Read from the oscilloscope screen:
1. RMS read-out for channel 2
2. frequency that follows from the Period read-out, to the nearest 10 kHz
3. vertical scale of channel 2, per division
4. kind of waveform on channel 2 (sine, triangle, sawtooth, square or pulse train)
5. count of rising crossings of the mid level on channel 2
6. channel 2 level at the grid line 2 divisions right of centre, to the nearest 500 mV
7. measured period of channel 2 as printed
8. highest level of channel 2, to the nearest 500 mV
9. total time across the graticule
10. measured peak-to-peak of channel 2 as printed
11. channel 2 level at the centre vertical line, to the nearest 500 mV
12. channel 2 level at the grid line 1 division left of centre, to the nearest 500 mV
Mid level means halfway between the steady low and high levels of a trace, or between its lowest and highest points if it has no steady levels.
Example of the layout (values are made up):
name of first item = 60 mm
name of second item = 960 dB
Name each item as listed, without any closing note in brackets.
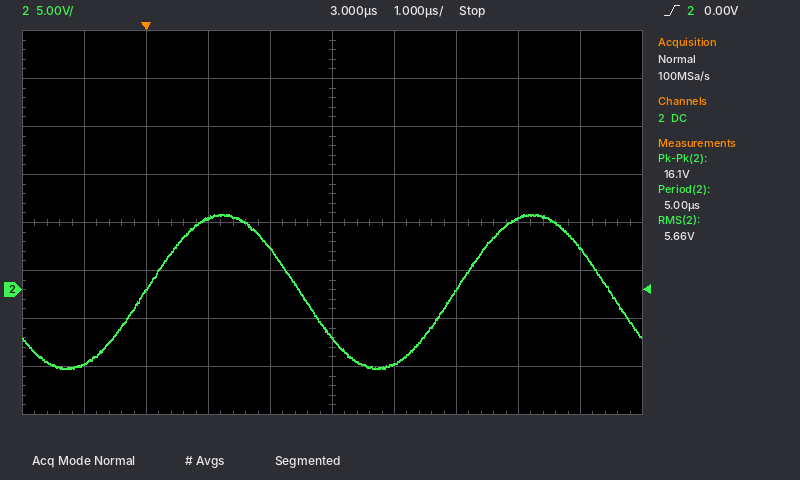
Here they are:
RMS read-out for channel 2 = 5.66 V
frequency that follows from the Period read-out, to the nearest 10 kHz = 200 kHz
vertical scale of channel 2, per division = 5 V
kind of waveform on channel 2 = sine
count of rising crossings of the mid level on channel 2 = 2
channel 2 level at the grid line 2 divisions right of centre, to the nearest 500 mV = 0.0 V
measured period of channel 2 as printed = 5.00 µs
highest level of channel 2, to the nearest 500 mV = 8.0 V
total time across the graticule = 10 µs
measured peak-to-peak of channel 2 as printed = 16.1 V
channel 2 level at the centre vertical line, to the nearest 500 mV = -5.0 V
channel 2 level at the grid line 1 division left of centre, to the nearest 500 mV = 4.5 V
